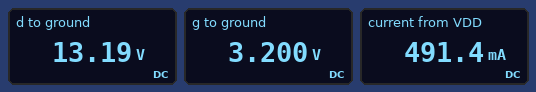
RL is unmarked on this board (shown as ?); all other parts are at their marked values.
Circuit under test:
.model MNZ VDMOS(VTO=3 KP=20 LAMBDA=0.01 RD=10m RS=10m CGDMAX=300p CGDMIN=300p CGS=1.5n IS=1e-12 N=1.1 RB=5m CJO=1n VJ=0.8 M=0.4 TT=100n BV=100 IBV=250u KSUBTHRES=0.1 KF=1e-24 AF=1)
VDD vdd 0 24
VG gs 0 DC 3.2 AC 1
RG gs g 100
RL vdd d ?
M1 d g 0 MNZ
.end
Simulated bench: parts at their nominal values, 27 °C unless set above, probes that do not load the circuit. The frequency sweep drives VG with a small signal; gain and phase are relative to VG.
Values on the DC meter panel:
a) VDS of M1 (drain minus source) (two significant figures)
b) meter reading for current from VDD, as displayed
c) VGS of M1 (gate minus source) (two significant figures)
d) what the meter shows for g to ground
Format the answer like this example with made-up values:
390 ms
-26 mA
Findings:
13 V
491.4 mA
3.2 V
3.200 V
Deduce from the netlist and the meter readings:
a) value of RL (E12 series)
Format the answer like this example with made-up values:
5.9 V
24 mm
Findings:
22 Ω
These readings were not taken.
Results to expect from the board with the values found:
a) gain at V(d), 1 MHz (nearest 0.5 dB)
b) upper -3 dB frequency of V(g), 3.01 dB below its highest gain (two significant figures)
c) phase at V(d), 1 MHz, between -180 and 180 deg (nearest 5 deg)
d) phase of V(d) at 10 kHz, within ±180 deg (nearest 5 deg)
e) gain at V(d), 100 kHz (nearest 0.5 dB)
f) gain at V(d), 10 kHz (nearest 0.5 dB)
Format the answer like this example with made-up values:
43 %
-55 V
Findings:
14.0 dB
62 kHz
95 deg
170 deg
32.5 dB
38.0 dB
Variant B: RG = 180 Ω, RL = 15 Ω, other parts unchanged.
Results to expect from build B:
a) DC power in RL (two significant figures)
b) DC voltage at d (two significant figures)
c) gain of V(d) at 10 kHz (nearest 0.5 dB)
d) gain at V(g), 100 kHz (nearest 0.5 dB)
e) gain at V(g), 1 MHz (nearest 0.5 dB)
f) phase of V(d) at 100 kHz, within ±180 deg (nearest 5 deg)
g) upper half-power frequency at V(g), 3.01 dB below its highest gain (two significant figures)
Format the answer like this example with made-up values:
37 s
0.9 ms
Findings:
3.8 W
16 V
35.0 dB
-7.5 dB
-26.5 dB
115 deg
46 kHz
